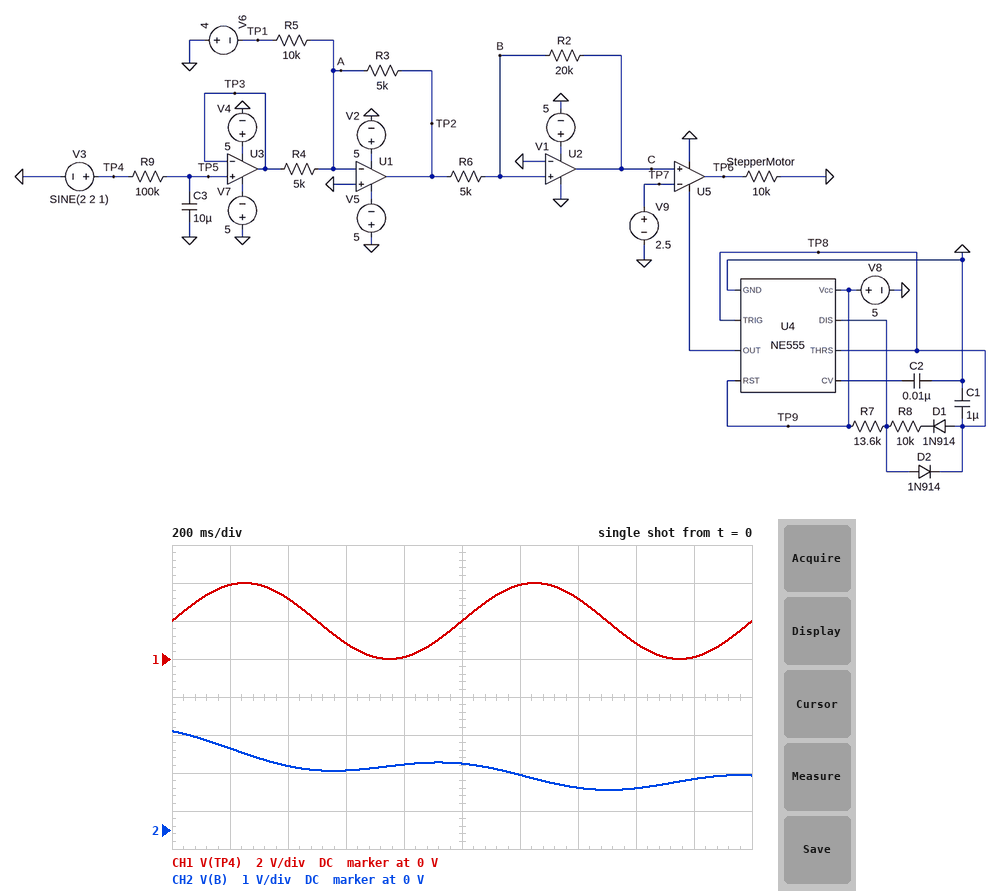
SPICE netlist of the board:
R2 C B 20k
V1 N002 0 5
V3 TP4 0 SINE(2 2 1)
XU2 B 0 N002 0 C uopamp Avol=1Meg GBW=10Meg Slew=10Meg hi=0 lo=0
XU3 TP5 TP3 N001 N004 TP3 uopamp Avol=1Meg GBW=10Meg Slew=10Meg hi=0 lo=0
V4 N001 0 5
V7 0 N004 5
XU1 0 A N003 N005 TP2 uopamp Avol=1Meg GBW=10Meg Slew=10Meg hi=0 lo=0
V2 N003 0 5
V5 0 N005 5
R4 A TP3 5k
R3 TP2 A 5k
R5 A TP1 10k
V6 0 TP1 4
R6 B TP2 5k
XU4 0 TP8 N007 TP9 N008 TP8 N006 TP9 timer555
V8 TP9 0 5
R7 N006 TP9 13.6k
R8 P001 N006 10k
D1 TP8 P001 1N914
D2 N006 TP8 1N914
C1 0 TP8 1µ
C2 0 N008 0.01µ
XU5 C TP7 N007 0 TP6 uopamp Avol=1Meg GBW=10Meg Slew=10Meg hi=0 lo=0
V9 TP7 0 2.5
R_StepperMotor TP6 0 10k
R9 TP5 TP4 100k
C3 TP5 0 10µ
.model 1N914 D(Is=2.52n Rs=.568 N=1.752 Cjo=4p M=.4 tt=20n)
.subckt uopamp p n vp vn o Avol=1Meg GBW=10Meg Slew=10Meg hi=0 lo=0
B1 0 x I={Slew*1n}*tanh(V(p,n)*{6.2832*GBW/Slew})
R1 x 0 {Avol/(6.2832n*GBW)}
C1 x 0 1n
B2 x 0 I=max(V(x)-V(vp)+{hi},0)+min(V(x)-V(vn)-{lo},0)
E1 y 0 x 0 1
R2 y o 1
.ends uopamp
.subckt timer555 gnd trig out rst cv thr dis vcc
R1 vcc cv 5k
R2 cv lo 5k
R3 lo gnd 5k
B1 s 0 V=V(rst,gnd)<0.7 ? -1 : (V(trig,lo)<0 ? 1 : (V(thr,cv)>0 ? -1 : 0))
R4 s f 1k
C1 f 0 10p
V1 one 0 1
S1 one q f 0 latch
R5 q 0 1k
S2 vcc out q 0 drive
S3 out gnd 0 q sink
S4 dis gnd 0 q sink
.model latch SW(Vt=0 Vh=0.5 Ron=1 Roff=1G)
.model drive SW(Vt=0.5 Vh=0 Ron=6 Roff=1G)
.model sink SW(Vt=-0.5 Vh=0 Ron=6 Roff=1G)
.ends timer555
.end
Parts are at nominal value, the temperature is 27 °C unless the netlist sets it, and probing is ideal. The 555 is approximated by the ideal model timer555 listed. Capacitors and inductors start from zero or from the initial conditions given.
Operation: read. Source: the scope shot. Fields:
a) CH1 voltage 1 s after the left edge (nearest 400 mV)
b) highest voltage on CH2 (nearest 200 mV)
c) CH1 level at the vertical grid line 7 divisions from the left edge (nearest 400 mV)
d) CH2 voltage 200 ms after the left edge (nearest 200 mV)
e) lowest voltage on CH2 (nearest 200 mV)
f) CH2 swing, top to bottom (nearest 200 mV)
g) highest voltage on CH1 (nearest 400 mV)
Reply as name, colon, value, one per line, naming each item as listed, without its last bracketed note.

CH1 voltage 1 s after the left edge: 2.0 V
highest voltage on CH2: 2.6 V
CH1 level at the vertical grid line 7 divisions from the left edge: 3.2 V
CH2 voltage 200 ms after the left edge: 2.2 V
lowest voltage on CH2: 1.0 V
CH2 swing, top to bottom: 1.6 V
highest voltage on CH1: 4.0 V
